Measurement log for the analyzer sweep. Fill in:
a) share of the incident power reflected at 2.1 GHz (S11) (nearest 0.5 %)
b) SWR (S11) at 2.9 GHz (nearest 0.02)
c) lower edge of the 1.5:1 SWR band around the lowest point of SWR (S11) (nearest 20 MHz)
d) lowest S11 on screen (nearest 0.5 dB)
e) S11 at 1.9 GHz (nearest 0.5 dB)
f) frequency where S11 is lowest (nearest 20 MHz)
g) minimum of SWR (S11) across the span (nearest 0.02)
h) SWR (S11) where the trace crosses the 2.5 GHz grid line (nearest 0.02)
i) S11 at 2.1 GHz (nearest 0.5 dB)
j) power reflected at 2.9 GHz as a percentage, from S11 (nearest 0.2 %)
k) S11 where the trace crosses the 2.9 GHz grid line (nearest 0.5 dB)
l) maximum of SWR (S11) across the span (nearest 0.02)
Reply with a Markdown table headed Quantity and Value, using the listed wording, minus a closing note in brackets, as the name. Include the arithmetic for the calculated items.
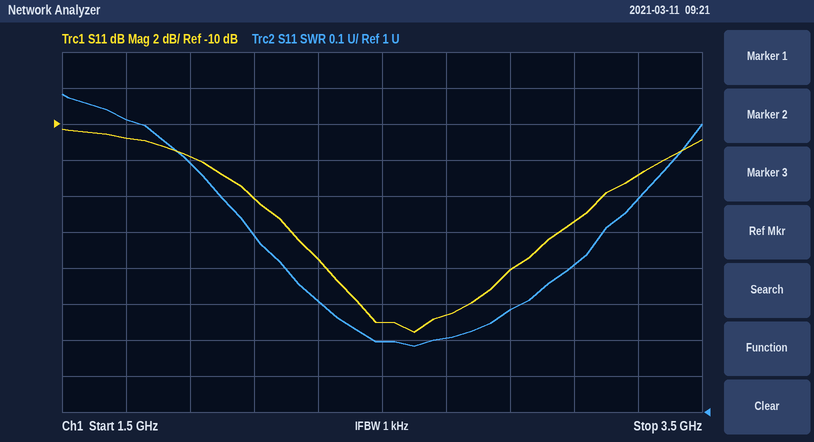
| Quantity | Value |
|---|---|
| share of the incident power reflected at 2.1 GHz (S11) | 10^(-14/10) ≈ 4.0 % |
| SWR (S11) at 2.9 GHz | 1.28 |
| lower edge of the 1.5:1 SWR band around the lowest point of SWR (S11) | 2.10 GHz |
| lowest S11 on screen | -21.5 dB |
| S11 at 1.9 GHz | -12.0 dB |
| frequency where S11 is lowest | 2.60 GHz |
| minimum of SWR (S11) across the span | 1.18 |
| SWR (S11) where the trace crosses the 2.5 GHz grid line | 1.20 |
| S11 at 2.1 GHz | -14.0 dB |
| power reflected at 2.9 GHz as a percentage, from S11 | 10^(-18/10) ≈ 1.6 % |
| S11 where the trace crosses the 2.9 GHz grid line | -18.0 dB |
| maximum of SWR (S11) across the span | 1.88 |
